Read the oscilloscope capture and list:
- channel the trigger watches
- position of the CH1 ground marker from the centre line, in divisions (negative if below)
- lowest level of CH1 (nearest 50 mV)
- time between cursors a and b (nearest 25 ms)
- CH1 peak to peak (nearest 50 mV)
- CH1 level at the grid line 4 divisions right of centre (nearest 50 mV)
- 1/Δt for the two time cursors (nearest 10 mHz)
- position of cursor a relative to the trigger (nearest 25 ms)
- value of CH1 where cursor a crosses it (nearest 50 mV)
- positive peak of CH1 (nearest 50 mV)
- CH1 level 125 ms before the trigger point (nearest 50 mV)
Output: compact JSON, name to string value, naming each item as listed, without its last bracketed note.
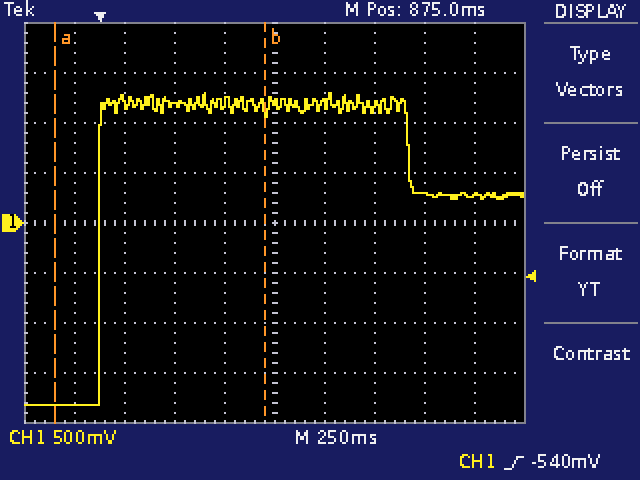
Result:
{"channel the trigger watches": "CH1", "position of the CH1 ground marker from the centre line, in divisions": "0.0 div", "lowest level of CH1": "-1.80 V", "time between cursors a and b": "1.050 s", "CH1 peak to peak": "3.10 V", "CH1 level at the grid line 4 divisions right of centre": "300 mV", "1/Δt for the two time cursors": "950 mHz", "position of cursor a relative to the trigger": "-225 ms", "value of CH1 where cursor a crosses it": "-1.80 V", "positive peak of CH1": "1.30 V", "CH1 level 125 ms before the trigger point": "-1.80 V"}
